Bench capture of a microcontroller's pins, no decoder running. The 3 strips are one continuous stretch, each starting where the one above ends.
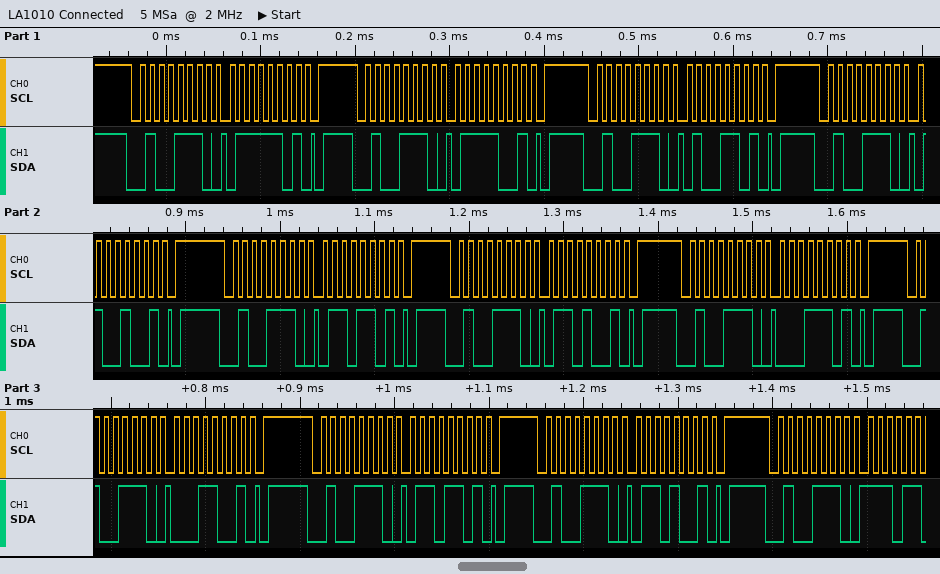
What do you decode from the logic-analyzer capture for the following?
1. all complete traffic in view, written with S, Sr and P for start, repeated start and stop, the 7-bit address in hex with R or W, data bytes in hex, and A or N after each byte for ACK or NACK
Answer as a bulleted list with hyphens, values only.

- S 27W A 7D A P S 27W A 79 A P S 27W A 4D A P S 27W A 49 A P S 27W A 6D A P S 27W A 69 A P S 27W A 1D A P S 27W A 19 A P S 27W A 6D A P S 27W A 69 A P S 27W A
